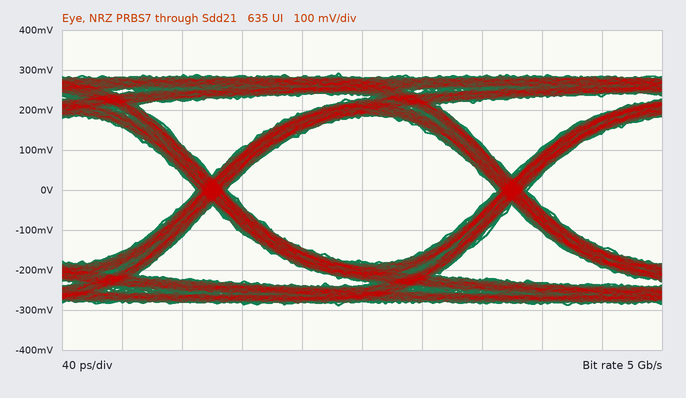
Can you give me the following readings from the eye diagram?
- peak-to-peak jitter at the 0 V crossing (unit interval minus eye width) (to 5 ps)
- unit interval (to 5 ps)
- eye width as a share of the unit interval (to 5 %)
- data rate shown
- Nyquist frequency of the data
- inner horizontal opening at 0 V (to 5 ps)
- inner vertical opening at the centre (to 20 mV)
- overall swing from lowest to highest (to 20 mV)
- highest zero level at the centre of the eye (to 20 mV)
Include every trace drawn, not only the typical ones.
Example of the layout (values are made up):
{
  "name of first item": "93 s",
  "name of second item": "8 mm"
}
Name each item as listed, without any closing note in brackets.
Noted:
{
  "peak-to-peak jitter at the 0 V crossing (unit interval minus eye width)": "20 ps",
  "unit interval": "200 ps",
  "eye width as a share of the unit interval": "90 %",
  "data rate shown": "5 Gb/s",
  "Nyquist frequency of the data": "2.5 GHz",
  "inner horizontal opening at 0 V": "180 ps",
  "inner vertical opening at the centre": "360 mV",
  "overall swing from lowest to highest": "580 mV",
  "highest zero level at the centre of the eye": "-180 mV"
}
